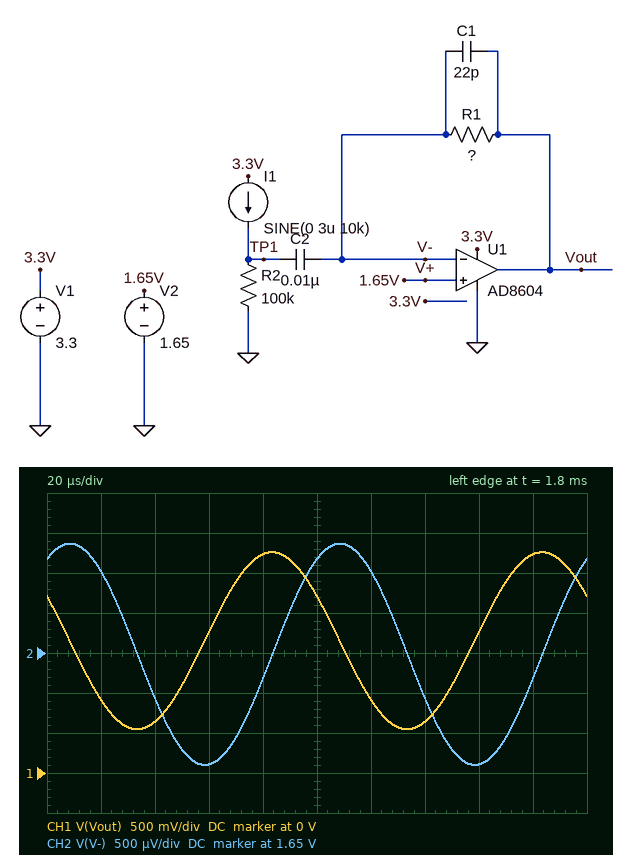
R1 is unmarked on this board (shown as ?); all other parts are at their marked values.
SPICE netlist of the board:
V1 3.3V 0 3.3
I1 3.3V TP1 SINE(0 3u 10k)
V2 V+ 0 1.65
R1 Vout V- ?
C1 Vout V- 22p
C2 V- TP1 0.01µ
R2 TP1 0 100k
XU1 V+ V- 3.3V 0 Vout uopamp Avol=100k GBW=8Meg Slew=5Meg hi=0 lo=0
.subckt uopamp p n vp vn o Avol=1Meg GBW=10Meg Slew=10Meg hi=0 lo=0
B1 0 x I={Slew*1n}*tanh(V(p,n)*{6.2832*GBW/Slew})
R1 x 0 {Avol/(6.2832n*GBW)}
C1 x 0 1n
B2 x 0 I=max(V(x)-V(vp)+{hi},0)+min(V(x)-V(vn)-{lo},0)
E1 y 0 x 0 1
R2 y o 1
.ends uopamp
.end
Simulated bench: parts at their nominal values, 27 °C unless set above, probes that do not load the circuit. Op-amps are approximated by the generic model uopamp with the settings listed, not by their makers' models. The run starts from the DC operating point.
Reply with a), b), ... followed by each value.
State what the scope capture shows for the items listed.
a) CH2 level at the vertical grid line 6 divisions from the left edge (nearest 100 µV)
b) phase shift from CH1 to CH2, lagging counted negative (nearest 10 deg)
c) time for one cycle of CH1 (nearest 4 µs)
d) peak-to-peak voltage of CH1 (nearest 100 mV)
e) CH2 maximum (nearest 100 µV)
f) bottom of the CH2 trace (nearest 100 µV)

a) 1.6510 V
b) -90 deg
c) 100 µs
d) 2.2 V
e) 1.6514 V
f) 1.6486 V
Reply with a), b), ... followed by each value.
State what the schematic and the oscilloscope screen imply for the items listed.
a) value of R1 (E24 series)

a) 430 kΩ
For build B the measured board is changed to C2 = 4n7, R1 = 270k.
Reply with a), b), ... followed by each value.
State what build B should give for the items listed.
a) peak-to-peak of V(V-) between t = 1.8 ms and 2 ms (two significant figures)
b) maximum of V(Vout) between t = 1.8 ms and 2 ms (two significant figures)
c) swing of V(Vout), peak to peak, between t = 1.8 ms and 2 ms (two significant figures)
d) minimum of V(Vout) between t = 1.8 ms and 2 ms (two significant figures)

a) 1.9 mV
b) 2.4 V
c) 1.5 V
d) 890 mV
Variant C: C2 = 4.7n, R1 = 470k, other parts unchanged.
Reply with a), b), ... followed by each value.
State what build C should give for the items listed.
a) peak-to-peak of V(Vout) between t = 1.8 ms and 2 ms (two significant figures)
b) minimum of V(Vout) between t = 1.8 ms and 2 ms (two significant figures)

a) 2.4 V
b) 470 mV
